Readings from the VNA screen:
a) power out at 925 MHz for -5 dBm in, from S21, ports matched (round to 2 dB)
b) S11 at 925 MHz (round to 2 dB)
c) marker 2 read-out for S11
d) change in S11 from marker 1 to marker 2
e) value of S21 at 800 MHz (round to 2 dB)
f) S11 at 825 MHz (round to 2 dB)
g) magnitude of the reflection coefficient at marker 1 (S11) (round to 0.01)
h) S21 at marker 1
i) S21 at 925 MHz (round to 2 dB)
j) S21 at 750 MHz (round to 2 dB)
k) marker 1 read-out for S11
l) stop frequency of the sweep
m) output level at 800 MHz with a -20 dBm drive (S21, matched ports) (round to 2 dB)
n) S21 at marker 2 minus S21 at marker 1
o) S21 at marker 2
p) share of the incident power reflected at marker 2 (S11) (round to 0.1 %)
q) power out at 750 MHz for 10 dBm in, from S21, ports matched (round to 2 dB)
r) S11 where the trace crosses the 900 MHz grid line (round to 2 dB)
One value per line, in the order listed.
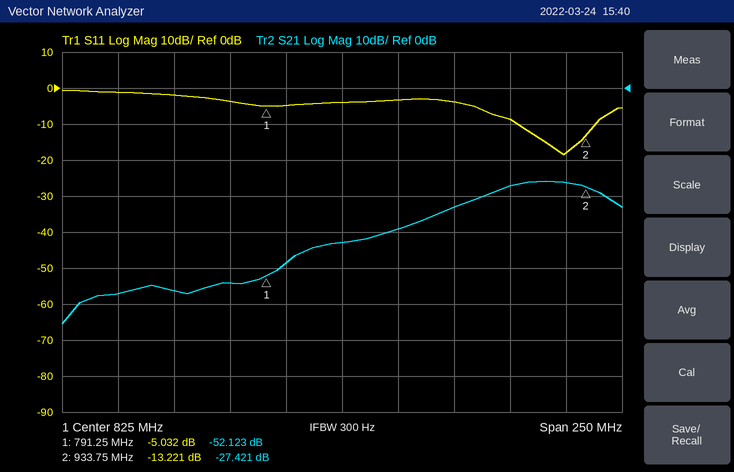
-32 dBm
-18 dB
-13.221 dB
-8.189 dB
-48 dB
-4 dB
0.56
-52.123 dB
-26 dB
-56 dB
-5.032 dB
950 MHz
-68 dBm
24.702 dB
-27.421 dB
4.8 %
-46 dBm
-8 dB
